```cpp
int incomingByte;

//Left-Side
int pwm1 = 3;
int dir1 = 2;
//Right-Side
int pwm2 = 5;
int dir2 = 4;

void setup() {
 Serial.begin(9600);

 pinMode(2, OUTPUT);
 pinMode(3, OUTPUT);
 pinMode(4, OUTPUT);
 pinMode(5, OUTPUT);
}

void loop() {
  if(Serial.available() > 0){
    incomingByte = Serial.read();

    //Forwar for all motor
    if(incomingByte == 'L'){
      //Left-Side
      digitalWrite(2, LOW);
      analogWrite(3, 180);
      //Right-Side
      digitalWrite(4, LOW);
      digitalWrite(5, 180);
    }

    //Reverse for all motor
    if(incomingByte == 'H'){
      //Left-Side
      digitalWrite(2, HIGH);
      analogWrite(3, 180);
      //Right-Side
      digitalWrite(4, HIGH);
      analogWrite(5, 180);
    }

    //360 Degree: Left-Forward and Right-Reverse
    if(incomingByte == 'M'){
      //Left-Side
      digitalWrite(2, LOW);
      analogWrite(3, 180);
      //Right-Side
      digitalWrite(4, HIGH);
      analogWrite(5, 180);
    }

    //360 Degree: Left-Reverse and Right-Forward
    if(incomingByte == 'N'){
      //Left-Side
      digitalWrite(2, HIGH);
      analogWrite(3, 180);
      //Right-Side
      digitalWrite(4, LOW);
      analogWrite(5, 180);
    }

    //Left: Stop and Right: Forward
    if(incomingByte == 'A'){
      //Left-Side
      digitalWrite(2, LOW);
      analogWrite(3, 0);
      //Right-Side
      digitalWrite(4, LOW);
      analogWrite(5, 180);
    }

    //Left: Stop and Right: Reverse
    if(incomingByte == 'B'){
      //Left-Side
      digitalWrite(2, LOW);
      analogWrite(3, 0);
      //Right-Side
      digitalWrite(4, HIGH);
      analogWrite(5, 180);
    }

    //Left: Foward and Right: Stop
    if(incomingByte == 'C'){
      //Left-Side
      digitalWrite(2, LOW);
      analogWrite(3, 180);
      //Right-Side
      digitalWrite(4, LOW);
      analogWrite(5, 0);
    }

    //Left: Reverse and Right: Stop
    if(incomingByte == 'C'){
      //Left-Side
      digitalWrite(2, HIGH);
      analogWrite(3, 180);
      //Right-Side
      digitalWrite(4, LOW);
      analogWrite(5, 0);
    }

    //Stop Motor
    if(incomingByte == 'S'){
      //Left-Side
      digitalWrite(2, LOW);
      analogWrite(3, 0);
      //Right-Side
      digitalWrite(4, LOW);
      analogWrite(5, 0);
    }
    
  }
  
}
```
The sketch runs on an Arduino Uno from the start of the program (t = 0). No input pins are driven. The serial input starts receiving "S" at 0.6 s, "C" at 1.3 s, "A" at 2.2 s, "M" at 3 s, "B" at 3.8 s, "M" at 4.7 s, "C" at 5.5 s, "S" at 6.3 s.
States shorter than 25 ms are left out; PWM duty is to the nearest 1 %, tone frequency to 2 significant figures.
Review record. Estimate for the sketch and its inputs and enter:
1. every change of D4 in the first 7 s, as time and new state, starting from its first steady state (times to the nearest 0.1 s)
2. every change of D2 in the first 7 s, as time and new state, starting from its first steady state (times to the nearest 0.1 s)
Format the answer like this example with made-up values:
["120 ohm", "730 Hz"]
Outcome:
["0 s low; 3 s high; 5.5 s low", "0 s low; 1.3 s high; 2.2 s low; 5.5 s high; 6.3 s low"]
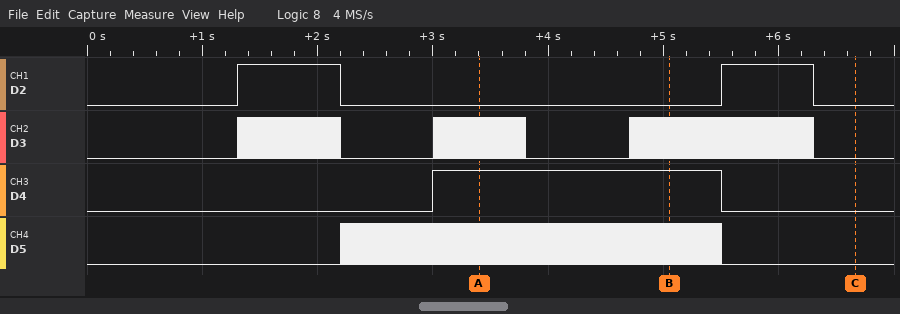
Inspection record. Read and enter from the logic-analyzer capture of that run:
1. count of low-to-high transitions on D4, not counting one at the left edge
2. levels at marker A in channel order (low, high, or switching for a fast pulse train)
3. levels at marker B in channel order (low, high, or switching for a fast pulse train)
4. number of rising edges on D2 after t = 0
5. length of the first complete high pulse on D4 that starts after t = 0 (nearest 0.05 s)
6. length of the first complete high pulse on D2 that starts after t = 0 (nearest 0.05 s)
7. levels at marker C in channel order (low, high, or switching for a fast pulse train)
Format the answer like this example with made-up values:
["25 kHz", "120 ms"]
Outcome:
["1", "D2 low, D3 switching, D4 high, D5 switching", "D2 low, D3 switching, D4 high, D5 switching", "2", "2.50 s", "0.90 s", "D2 low, D3 low, D4 low, D5 low"]
